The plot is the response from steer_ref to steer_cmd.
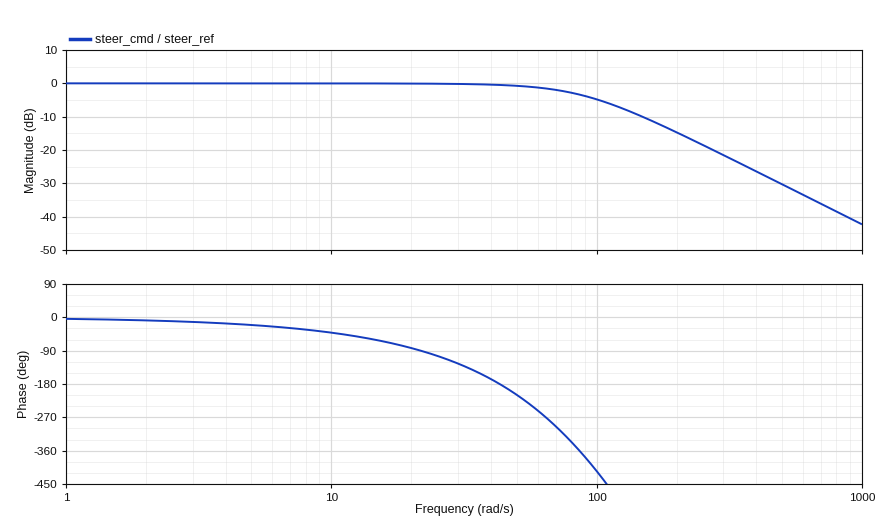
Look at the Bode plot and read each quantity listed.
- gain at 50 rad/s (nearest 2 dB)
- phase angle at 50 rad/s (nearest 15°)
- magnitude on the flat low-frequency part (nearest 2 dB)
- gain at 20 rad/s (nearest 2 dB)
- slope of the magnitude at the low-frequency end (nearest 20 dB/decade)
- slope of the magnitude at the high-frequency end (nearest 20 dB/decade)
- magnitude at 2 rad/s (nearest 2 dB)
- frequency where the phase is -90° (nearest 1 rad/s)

0 dB
-210°
0 dB
0 dB
0 dB/decade
-40 dB/decade
0 dB
22 rad/s
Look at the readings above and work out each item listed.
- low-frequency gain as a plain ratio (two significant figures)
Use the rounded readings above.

1.0
